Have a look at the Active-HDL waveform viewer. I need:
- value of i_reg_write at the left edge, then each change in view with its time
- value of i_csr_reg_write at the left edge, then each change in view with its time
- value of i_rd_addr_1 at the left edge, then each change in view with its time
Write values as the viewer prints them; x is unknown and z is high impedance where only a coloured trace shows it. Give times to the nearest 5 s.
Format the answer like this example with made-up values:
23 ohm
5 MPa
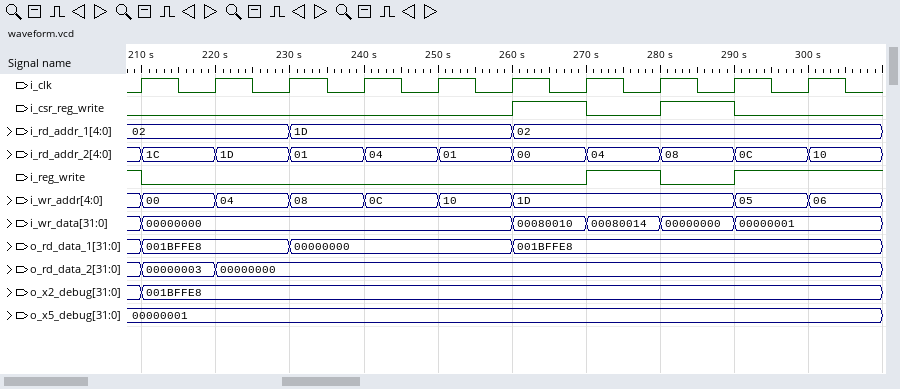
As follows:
1, 0 at 210 s, 1 at 270 s, 0 at 280 s, 1 at 290 s
0, 1 at 260 s, 0 at 270 s, 1 at 280 s, 0 at 290 s
02, 1D at 230 s, 02 at 260 s
